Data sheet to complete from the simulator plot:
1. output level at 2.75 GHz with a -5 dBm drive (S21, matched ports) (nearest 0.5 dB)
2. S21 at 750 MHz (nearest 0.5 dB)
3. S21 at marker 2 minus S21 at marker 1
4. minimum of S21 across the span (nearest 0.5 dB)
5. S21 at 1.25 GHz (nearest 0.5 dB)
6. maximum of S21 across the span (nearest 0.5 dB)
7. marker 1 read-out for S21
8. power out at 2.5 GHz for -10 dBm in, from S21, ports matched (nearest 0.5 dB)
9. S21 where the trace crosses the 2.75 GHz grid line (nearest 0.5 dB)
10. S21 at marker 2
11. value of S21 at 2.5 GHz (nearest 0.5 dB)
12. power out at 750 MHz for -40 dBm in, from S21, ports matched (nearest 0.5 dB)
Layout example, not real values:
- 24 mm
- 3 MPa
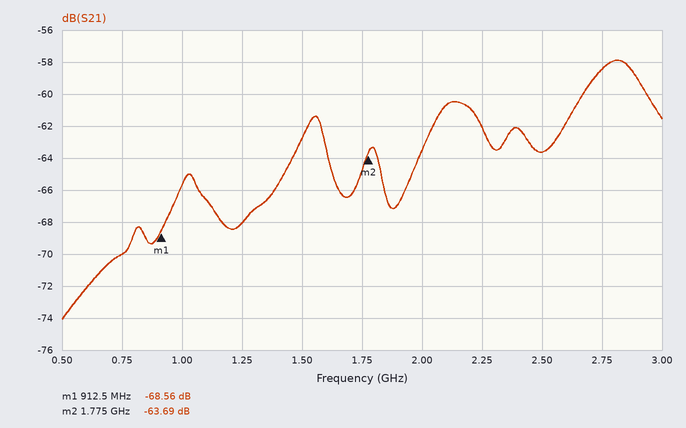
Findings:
- -63.5 dBm
- -70.0 dB
- 4.87 dB
- -74.0 dB
- -68.0 dB
- -58.0 dB
- -68.56 dB
- -73.5 dBm
- -58.5 dB
- -63.69 dB
- -63.5 dB
- -110.0 dBm
